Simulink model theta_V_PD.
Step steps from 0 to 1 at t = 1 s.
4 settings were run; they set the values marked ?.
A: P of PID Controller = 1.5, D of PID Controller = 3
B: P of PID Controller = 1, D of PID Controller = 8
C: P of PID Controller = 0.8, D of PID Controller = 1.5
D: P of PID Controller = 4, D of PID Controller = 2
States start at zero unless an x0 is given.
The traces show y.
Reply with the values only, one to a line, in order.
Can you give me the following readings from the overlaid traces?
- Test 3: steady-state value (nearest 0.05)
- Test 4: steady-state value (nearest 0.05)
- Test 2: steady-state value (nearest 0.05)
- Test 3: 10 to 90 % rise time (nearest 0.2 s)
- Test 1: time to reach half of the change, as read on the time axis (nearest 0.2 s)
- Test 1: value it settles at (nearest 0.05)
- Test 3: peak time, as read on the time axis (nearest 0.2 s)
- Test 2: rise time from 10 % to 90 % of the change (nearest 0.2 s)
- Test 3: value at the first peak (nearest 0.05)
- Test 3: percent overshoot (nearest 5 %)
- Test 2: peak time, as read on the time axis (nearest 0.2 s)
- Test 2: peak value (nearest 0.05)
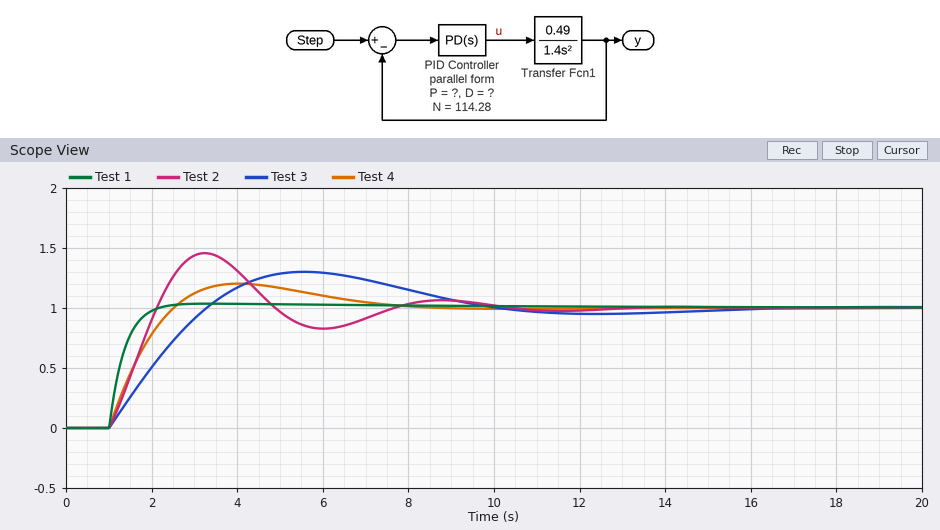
1.00
1.00
1.00
1.8 s
1.2 s
1.00
5.6 s
0.8 s
1.30
30 %
3.2 s
1.45
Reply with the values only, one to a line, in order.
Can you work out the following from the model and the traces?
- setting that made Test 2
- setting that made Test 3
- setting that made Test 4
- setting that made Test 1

D
C
A
B
